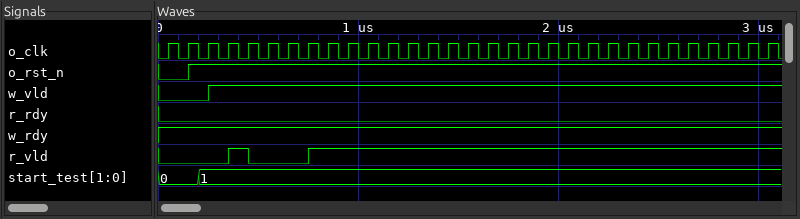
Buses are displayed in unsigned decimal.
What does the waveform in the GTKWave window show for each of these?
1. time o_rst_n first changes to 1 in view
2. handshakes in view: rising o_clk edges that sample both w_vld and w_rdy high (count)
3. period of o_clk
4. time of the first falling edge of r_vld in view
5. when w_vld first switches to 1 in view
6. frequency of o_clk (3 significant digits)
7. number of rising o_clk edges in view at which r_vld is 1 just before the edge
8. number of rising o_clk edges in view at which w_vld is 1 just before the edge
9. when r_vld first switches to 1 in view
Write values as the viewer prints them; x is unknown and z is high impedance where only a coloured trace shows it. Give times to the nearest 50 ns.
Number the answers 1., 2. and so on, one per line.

1. 150 ns
2. 28
3. 100 ns
4. 450 ns
5. 250 ns
6. 10.0 MHz
7. 24
8. 28
9. 350 ns
